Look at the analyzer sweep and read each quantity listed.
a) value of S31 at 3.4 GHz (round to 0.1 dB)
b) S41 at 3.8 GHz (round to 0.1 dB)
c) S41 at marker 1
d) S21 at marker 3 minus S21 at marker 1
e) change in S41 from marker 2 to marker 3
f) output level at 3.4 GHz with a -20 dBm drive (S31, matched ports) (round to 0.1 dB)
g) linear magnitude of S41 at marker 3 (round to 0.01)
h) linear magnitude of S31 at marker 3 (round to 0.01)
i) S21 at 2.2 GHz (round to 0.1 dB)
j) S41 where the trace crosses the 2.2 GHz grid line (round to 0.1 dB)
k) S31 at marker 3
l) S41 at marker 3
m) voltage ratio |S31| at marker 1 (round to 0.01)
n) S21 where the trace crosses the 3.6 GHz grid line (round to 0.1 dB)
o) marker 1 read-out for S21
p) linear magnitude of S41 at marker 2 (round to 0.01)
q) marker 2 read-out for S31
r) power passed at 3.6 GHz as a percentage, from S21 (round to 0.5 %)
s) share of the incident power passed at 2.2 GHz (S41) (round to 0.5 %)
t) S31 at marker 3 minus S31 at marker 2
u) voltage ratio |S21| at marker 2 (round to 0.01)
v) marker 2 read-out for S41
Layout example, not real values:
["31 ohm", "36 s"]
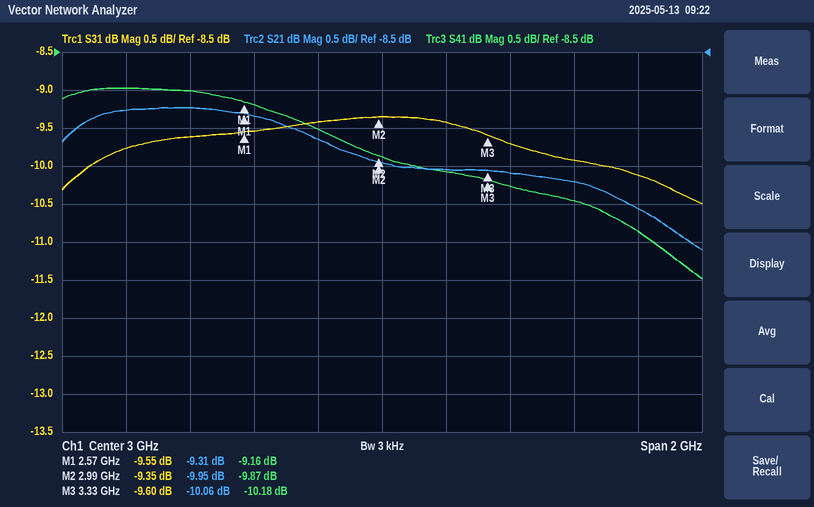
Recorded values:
["-9.7 dB", "-10.9 dB", "-9.16 dB", "-0.75 dB", "-0.31 dB", "-29.7 dBm", "0.31", "0.33", "-9.3 dB", "-9.0 dB", "-9.60 dB", "-10.18 dB", "0.33", "-10.2 dB", "-9.31 dB", "0.32", "-9.35 dB", "9.5 %", "12.5 %", "-0.25 dB", "0.32", "-9.87 dB"]
